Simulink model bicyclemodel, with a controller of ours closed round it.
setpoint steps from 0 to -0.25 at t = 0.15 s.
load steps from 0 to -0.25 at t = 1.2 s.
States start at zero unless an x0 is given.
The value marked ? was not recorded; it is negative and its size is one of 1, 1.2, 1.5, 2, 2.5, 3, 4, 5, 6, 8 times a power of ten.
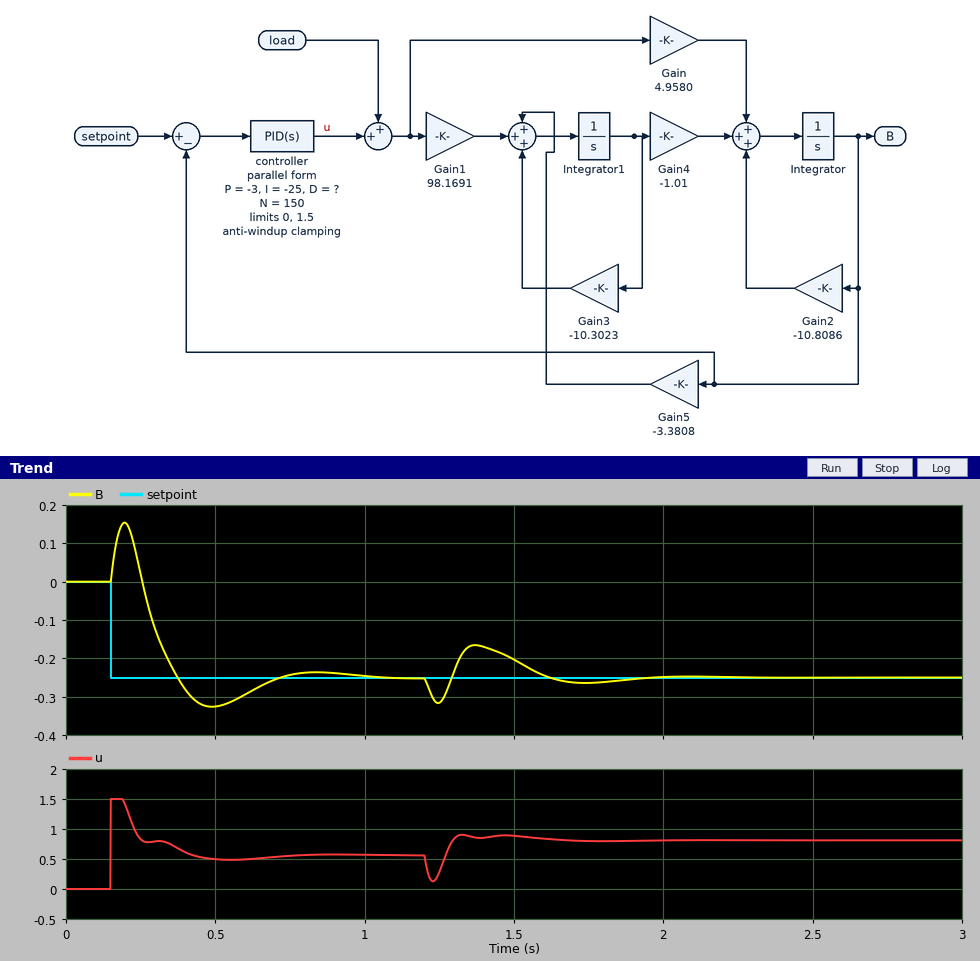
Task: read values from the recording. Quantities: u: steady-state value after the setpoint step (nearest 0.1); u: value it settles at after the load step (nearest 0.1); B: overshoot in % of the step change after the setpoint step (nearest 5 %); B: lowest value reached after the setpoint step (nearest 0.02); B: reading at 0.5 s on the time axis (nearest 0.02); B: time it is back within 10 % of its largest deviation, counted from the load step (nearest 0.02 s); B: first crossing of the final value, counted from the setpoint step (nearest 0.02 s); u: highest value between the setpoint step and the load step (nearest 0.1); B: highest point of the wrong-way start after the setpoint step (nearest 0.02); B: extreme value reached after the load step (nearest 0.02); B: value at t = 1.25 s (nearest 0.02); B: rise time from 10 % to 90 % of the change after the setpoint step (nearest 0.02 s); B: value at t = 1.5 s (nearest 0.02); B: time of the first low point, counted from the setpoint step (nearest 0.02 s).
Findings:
0.6
0.8
30 %
-0.32
-0.32
0.64 s
0.22 s
1.5
0.16
-0.16
-0.32
0.10 s
-0.20
0.34 s
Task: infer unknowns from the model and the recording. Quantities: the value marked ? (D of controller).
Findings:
-0.15
